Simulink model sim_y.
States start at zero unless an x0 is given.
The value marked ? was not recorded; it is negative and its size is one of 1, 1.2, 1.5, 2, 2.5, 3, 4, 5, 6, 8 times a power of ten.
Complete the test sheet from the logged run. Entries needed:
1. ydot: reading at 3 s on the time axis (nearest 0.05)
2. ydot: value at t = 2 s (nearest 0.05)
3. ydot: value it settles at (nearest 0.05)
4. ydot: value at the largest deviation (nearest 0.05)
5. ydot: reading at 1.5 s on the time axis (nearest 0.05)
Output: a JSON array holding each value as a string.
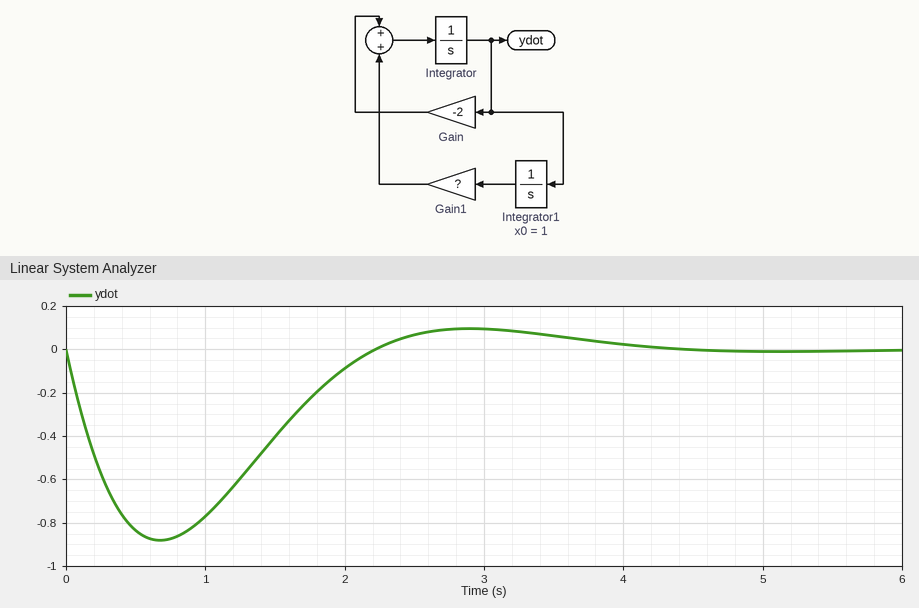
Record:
["0.10", "-0.10", "0.00", "-0.90", "-0.40"]
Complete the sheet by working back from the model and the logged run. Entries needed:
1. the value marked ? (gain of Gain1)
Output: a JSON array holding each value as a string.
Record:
["-3"]
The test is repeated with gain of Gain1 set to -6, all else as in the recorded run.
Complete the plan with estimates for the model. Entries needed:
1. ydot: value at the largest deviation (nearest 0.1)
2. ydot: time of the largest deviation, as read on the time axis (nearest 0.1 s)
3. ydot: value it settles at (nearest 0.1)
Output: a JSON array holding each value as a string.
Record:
["-1.5", "0.5 s", "0.0"]
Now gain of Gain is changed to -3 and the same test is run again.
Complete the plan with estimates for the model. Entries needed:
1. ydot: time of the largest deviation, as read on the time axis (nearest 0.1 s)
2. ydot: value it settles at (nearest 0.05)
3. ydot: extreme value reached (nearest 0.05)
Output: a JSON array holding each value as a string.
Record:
["0.6 s", "0.00", "-0.70"]
